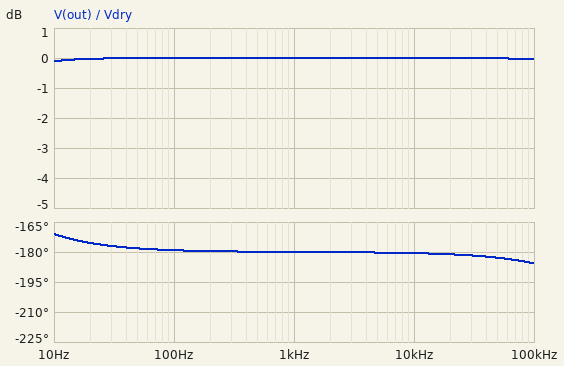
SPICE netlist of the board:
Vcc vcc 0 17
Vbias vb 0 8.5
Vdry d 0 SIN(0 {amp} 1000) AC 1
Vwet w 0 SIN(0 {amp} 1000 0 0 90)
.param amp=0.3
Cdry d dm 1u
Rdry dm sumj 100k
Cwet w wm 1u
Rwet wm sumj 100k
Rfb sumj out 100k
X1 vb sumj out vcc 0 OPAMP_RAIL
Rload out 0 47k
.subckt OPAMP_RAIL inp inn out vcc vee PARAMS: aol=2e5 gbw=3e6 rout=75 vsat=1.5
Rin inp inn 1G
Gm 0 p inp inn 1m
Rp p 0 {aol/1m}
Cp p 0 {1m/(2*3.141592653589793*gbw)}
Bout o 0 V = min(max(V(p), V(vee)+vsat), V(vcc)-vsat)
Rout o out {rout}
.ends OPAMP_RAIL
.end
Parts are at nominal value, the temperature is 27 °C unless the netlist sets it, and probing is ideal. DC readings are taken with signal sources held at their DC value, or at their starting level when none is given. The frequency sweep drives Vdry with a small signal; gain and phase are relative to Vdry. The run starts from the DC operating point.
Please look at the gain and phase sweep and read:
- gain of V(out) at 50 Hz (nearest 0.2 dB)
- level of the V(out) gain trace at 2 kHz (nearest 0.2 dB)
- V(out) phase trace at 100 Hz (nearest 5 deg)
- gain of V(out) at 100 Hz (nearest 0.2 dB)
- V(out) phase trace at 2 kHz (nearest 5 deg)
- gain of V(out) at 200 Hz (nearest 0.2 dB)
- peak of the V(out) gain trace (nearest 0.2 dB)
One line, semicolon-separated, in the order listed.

0 dB; 0 dB; -180 deg; 0 dB; -180 deg; 0 dB; 0 dB
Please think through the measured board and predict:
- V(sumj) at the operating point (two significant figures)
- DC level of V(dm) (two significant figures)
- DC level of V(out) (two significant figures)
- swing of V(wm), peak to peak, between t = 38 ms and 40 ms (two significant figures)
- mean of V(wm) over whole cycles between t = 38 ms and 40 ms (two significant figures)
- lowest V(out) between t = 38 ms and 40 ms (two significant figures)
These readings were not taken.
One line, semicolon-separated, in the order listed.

8.5 V; 8.5 V; 8.5 V; 600 mV; 8.3 V; 8.3 V
